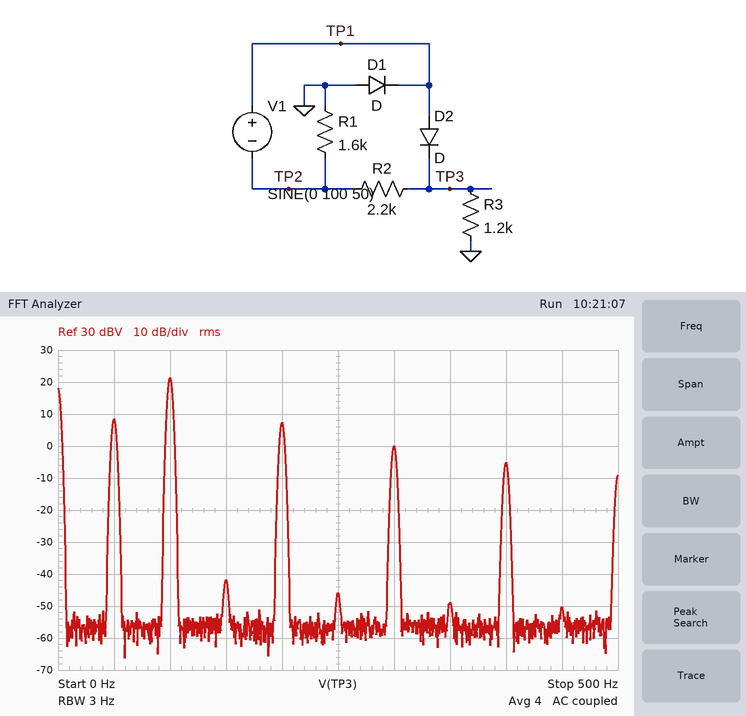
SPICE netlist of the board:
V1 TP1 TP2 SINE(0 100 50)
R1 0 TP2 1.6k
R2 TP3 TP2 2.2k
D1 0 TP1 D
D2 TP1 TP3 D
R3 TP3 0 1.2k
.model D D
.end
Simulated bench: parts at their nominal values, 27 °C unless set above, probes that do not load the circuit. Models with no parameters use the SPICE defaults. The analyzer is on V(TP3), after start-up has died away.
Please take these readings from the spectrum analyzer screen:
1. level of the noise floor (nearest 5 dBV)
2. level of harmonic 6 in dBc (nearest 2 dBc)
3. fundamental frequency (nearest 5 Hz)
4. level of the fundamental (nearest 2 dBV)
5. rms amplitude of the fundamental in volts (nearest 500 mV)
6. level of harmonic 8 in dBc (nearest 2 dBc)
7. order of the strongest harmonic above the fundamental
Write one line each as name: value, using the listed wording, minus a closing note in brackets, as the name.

level of the noise floor: -55 dBV
level of harmonic 6 in dBc: -8 dBc
fundamental frequency: 50 Hz
level of the fundamental: 8 dBV
rms amplitude of the fundamental in volts: 2.5 V
level of harmonic 8 in dBc: -14 dBc
order of the strongest harmonic above the fundamental: 2
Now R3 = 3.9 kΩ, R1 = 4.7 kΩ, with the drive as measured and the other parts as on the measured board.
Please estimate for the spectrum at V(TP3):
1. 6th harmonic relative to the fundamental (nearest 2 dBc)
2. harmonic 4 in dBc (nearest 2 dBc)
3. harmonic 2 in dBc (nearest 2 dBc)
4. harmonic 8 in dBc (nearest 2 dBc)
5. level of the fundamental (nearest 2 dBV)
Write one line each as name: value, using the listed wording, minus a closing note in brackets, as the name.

6th harmonic relative to the fundamental: -14 dBc
harmonic 4 in dBc: -6 dBc
harmonic 2 in dBc: 8 dBc
harmonic 8 in dBc: -18 dBc
level of the fundamental: 16 dBV
